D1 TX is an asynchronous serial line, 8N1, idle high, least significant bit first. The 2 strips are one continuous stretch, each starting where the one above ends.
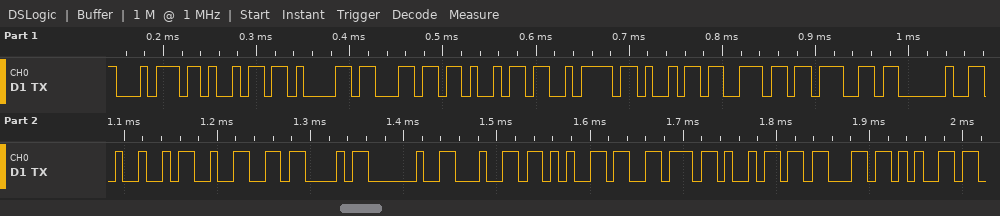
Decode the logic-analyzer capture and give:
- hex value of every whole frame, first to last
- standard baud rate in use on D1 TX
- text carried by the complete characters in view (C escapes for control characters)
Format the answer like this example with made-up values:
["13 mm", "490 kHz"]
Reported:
["0x74 0x69 0x61 0x6C 0x69 0x7A 0x69 0x6E 0x67 0x20 0x49 0x32 0x43 0x20 0x64 0x65 0x76 0x69 0x63 0x65", "115200 baud", "\"tializing I2C device\""]
